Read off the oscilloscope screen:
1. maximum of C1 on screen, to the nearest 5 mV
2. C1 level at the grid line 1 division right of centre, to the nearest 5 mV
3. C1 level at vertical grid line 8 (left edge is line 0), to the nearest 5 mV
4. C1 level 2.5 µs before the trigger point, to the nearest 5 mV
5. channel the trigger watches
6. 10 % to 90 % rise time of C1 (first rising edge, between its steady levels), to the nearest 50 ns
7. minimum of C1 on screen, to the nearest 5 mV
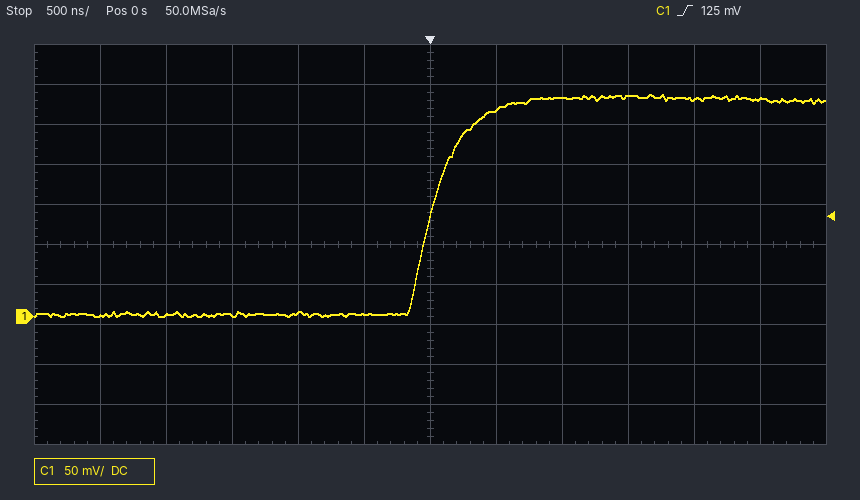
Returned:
280 mV
260 mV
275 mV
0 mV
C1
500 ns
0 mV
